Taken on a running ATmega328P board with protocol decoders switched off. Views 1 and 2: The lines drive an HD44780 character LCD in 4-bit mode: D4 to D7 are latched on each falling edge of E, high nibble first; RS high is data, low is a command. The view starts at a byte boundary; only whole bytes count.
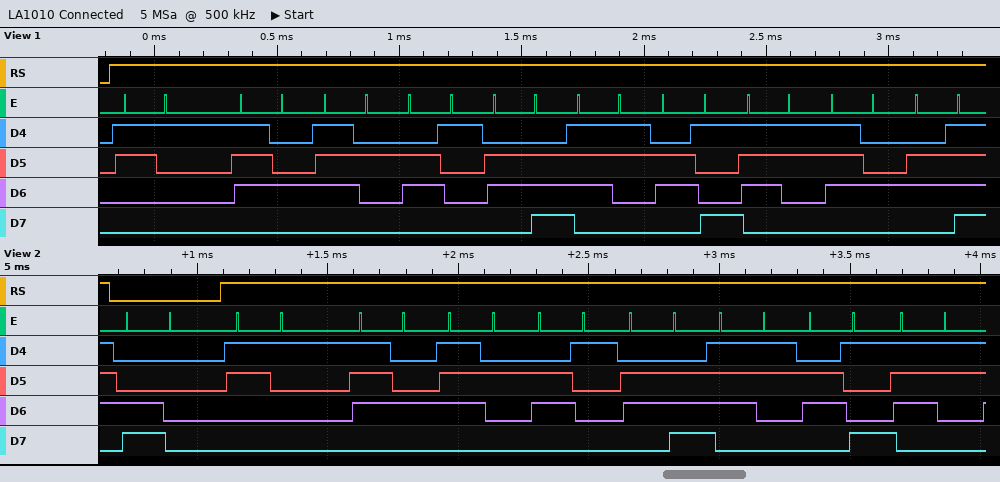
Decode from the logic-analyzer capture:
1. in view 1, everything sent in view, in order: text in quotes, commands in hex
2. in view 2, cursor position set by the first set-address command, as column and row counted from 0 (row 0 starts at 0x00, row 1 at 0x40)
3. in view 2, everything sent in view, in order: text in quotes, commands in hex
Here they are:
"1transisto"
column 0, row 1
0xC0 "1transis"
